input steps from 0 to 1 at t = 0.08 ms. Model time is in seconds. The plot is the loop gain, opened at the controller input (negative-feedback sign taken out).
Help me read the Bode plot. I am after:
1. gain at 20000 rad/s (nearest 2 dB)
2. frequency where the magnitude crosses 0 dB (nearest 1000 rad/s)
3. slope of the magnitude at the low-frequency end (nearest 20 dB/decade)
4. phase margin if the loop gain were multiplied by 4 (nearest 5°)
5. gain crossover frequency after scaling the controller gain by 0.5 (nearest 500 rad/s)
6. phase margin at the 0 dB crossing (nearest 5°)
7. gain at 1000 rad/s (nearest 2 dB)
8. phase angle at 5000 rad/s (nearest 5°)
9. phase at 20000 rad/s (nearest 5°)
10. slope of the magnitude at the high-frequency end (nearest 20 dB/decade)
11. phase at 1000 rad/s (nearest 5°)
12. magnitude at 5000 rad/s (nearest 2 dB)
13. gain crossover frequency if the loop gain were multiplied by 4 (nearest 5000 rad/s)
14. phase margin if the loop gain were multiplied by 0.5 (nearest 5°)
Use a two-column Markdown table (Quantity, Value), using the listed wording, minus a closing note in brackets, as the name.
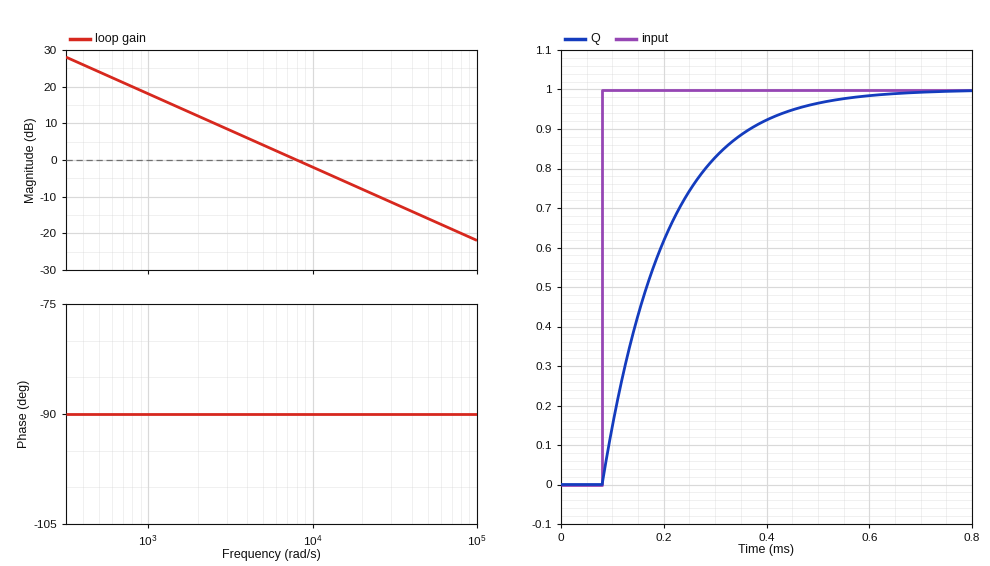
| Quantity | Value |
|---|---|
| gain at 20000 rad/s | -8 dB |
| frequency where the magnitude crosses 0 dB | 8000 rad/s |
| slope of the magnitude at the low-frequency end | -20 dB/decade |
| phase margin if the loop gain were multiplied by 4 | 90° |
| gain crossover frequency after scaling the controller gain by 0.5 | 4000 rad/s |
| phase margin at the 0 dB crossing | 90° |
| gain at 1000 rad/s | 18 dB |
| phase angle at 5000 rad/s | -90° |
| phase at 20000 rad/s | -90° |
| slope of the magnitude at the high-frequency end | -20 dB/decade |
| phase at 1000 rad/s | -90° |
| magnitude at 5000 rad/s | 4 dB |
| gain crossover frequency if the loop gain were multiplied by 4 | 30000 rad/s |
| phase margin if the loop gain were multiplied by 0.5 | 90° |
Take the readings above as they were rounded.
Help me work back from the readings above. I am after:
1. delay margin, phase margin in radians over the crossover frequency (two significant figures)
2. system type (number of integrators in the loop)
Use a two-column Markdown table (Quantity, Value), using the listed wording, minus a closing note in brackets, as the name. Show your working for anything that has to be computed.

| Quantity | Value |
|---|---|
| delay margin, phase margin in radians over the crossover frequency | 90 × π / 180 / 8000 = 0.00020 s |
| system type | 1 |
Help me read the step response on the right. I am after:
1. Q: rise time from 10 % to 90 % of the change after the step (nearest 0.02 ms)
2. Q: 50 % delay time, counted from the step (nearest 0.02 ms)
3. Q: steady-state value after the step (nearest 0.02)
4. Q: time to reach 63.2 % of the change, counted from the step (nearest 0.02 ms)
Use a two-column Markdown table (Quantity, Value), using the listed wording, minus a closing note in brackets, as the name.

| Quantity | Value |
|---|---|
| Q: rise time from 10 % to 90 % of the change after the step | 0.28 ms |
| Q: 50 % delay time, counted from the step | 0.08 ms |
| Q: steady-state value after the step | 1.00 |
| Q: time to reach 63.2 % of the change, counted from the step | 0.12 ms |
